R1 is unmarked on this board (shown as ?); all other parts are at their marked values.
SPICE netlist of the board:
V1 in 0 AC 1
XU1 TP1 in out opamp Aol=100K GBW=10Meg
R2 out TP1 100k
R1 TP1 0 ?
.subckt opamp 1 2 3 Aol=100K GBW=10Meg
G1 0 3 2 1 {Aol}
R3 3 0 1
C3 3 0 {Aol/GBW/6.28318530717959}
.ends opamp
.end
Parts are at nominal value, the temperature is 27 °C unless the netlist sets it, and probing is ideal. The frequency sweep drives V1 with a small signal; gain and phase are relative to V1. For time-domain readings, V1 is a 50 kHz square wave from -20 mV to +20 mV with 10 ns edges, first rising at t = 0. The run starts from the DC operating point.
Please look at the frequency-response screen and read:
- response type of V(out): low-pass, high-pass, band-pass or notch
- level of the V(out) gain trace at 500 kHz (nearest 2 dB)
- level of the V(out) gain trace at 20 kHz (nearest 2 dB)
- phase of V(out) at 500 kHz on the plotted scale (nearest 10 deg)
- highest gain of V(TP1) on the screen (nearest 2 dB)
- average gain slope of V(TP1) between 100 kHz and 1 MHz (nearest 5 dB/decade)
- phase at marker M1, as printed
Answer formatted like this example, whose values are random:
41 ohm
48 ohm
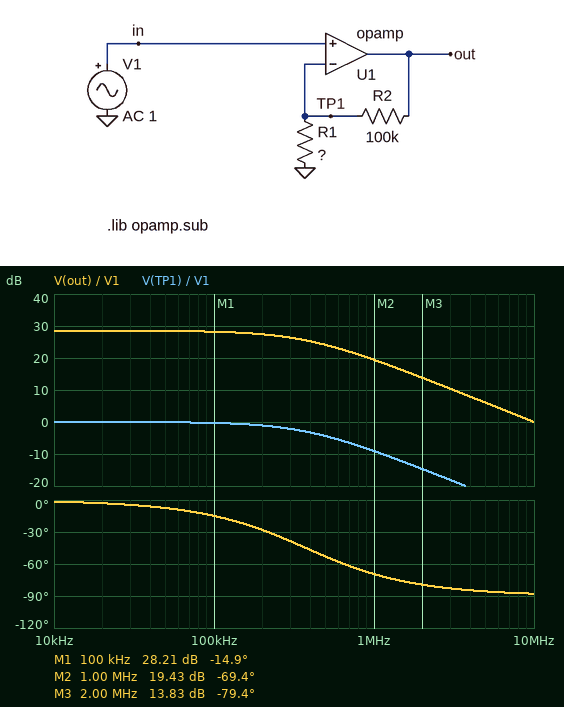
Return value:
low-pass
24 dB
28 dB
-50 deg
0 dB
-10 dB/decade
-14.9 deg
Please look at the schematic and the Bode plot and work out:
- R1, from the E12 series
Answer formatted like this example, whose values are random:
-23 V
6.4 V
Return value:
3.9 kΩ
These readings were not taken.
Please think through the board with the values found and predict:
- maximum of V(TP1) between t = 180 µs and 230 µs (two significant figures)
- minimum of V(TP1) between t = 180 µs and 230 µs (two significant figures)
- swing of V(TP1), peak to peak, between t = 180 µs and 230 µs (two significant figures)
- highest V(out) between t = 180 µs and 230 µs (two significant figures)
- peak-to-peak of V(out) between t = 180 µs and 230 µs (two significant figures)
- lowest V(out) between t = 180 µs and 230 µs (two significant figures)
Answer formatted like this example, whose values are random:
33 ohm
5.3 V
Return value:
20 mV
-20 mV
40 mV
530 mV
1.1 V
-530 mV
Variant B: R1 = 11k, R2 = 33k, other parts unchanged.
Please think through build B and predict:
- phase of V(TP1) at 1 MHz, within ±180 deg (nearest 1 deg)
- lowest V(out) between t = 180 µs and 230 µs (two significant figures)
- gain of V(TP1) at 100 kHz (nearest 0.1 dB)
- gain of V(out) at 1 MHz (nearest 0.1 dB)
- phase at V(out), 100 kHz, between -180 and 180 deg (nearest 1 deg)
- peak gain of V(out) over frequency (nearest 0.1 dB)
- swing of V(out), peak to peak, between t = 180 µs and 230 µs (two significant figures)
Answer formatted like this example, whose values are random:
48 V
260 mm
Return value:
-22 deg
-80 mV
0 dB
11.4 dB
-2 deg
12.0 dB
160 mV
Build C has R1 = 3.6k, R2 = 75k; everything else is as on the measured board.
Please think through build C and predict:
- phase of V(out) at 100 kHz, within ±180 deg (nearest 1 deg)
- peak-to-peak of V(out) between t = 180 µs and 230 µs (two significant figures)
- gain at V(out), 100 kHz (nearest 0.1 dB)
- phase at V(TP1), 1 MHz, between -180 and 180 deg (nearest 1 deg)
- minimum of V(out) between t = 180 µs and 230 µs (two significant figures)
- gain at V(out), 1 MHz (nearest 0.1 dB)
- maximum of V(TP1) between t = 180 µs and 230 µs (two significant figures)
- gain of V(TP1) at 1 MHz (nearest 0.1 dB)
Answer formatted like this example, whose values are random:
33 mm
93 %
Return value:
-12 deg
870 mV
26.6 dB
-65 deg
-440 mV
19.2 dB
20 mV
-7.6 dB
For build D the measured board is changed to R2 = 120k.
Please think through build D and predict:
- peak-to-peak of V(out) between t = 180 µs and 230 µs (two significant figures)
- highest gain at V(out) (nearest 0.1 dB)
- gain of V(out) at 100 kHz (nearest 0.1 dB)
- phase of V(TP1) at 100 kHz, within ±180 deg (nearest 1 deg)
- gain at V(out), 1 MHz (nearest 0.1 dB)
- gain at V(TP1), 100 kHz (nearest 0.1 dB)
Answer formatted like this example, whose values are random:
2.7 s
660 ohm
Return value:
1.3 V
30.0 dB
29.6 dB
-18 deg
19.6 dB
-0.4 dB
